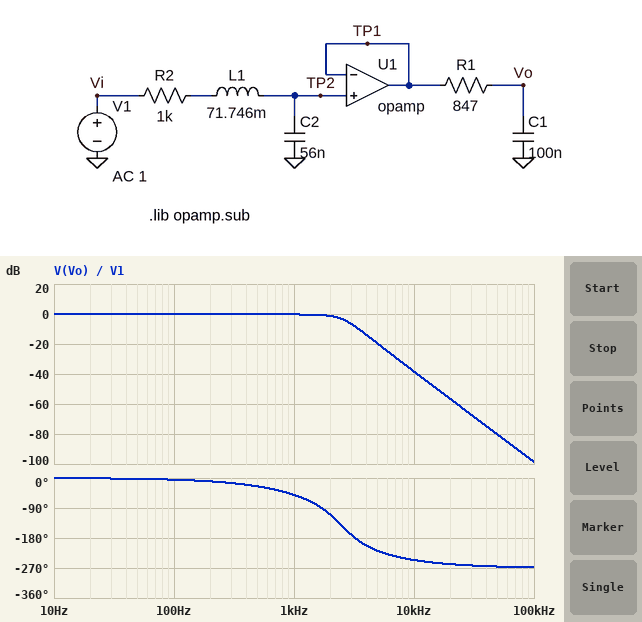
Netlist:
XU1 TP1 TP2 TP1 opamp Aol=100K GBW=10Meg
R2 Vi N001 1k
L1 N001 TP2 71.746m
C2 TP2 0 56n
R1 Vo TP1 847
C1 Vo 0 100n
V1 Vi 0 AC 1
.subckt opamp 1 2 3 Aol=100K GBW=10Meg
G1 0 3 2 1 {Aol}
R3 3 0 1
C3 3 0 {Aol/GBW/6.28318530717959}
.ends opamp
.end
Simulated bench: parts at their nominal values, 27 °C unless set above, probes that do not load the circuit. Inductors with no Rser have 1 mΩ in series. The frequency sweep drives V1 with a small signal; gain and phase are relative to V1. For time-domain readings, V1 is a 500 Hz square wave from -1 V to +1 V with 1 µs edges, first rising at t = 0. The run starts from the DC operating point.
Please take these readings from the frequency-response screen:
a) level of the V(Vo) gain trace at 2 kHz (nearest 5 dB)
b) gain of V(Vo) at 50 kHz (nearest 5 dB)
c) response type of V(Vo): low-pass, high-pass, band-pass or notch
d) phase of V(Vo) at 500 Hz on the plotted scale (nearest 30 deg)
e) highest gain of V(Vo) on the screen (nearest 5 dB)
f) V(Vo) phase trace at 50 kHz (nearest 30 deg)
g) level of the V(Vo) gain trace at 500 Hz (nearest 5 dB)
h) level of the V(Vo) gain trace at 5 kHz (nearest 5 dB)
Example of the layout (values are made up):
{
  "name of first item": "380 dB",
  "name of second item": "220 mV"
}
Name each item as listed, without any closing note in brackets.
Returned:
{
  "level of the V(Vo) gain trace at 2 kHz": "0 dB",
  "gain of V(Vo) at 50 kHz": "-80 dB",
  "response type of V(Vo): low-pass, high-pass, band-pass or notch": "low-pass",
  "phase of V(Vo) at 500 Hz on the plotted scale": "-30 deg",
  "highest gain of V(Vo) on the screen": "0 dB",
  "V(Vo) phase trace at 50 kHz": "-270 deg",
  "level of the V(Vo) gain trace at 500 Hz": "0 dB",
  "level of the V(Vo) gain trace at 5 kHz": "-20 dB"
}
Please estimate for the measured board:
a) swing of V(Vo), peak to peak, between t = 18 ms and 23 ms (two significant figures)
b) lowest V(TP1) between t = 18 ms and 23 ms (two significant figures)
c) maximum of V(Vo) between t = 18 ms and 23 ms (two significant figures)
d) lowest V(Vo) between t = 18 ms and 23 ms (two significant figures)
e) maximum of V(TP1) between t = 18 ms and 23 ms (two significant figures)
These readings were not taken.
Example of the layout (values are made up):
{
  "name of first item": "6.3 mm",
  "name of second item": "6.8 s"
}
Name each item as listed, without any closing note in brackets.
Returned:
{
  "swing of V(Vo), peak to peak, between t = 18 ms and 23 ms": "2.3 V",
  "lowest V(TP1) between t = 18 ms and 23 ms": "-1.4 V",
  "maximum of V(Vo) between t = 18 ms and 23 ms": "1.1 V",
  "lowest V(Vo) between t = 18 ms and 23 ms": "-1.1 V",
  "maximum of V(TP1) between t = 18 ms and 23 ms": "1.4 V"
}
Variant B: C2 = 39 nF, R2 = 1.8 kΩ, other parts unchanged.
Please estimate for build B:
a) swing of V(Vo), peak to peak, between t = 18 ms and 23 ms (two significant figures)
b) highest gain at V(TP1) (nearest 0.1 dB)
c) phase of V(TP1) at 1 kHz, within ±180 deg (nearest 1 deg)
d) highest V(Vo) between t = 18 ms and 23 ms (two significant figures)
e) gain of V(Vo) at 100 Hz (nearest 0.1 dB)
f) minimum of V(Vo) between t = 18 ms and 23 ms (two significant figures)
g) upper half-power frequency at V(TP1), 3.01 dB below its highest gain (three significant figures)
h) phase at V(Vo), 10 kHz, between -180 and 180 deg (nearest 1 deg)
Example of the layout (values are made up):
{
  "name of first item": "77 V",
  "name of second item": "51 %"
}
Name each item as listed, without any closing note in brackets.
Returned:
{
  "swing of V(Vo), peak to peak, between t = 18 ms and 23 ms": "2.0 V",
  "highest gain at V(TP1)": "0.1 dB",
  "phase of V(TP1) at 1 kHz, within ±180 deg": "-26 deg",
  "highest V(Vo) between t = 18 ms and 23 ms": "1.0 V",
  "gain of V(Vo) at 100 Hz": "0 dB",
  "minimum of V(Vo) between t = 18 ms and 23 ms": "-1.0 V",
  "upper half-power frequency at V(TP1), 3.01 dB below its highest gain": "3.17 kHz",
  "phase at V(Vo), 10 kHz, between -180 and 180 deg": "124 deg"
}
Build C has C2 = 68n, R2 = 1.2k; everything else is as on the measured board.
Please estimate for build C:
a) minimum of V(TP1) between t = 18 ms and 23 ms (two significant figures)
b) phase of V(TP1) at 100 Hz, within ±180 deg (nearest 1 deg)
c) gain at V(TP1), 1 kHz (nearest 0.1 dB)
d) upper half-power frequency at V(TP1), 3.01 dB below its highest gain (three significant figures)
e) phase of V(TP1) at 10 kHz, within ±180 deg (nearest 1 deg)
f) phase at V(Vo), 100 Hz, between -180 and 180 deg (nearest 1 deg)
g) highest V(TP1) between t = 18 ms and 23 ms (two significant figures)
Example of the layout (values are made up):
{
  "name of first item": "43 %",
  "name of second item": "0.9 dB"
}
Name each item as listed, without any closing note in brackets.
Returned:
{
  "minimum of V(TP1) between t = 18 ms and 23 ms": "-1.2 V",
  "phase of V(TP1) at 100 Hz, within ±180 deg": "-3 deg",
  "gain at V(TP1), 1 kHz": "0.4 dB",
  "upper half-power frequency at V(TP1), 3.01 dB below its highest gain": "2.56 kHz",
  "phase of V(TP1) at 10 kHz, within ±180 deg": "-164 deg",
  "phase at V(Vo), 100 Hz, between -180 and 180 deg": "-6 deg",
  "highest V(TP1) between t = 18 ms and 23 ms": "1.2 V"
}
